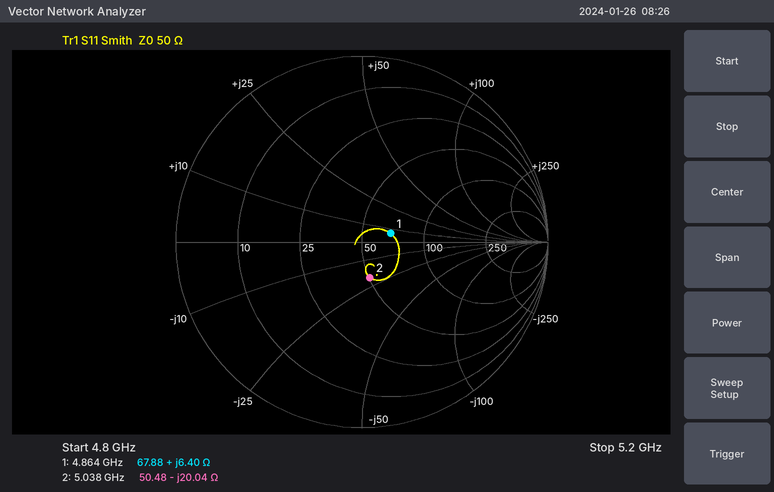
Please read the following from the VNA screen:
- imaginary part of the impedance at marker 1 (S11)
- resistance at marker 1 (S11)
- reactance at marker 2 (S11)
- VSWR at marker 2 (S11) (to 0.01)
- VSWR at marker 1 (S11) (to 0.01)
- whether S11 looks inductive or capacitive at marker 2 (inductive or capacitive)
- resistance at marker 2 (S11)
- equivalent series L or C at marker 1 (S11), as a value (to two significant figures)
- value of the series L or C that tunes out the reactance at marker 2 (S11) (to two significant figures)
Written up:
+6.40 Ω
67.88 Ω
-20.04 Ω
1.49
1.38
capacitive
50.48 Ω
210 pH
630 pH
